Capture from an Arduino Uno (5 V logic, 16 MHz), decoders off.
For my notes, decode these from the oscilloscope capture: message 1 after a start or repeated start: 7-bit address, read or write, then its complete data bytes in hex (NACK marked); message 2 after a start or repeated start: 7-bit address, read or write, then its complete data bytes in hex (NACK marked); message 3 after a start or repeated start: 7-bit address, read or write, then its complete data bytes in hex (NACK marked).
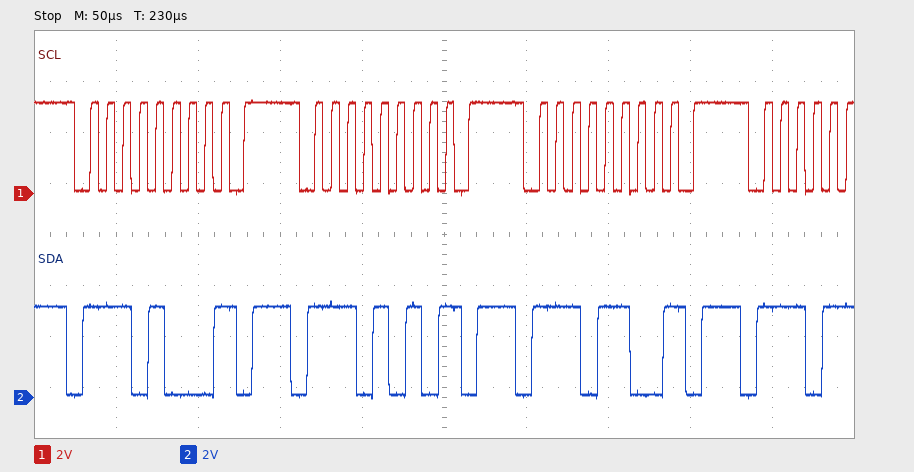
0x74 write NACK
0x75 write NACK
0x76 write NACK
